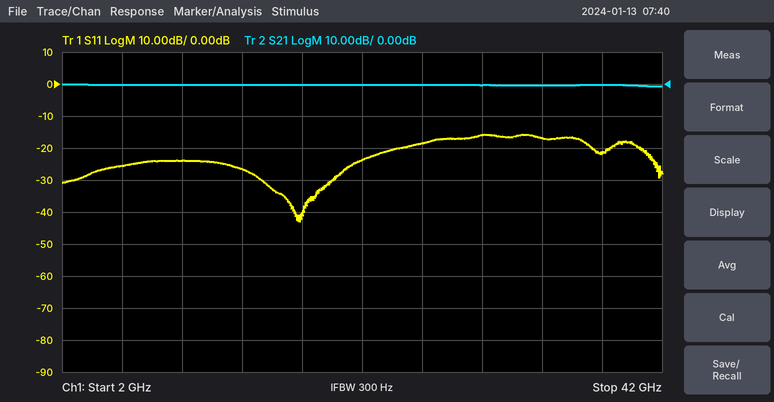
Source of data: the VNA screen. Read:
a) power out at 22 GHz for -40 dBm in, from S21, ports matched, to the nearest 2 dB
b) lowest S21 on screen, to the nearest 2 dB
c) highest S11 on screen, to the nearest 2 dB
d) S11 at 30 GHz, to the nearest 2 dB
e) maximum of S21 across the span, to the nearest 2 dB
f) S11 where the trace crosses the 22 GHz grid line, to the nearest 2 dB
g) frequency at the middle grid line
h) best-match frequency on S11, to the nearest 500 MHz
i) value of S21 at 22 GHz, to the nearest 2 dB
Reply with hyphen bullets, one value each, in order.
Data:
- -40 dBm
- 0 dB
- -16 dB
- -16 dB
- 0 dB
- -24 dB
- 22 GHz
- 18.0 GHz
- 0 dB
